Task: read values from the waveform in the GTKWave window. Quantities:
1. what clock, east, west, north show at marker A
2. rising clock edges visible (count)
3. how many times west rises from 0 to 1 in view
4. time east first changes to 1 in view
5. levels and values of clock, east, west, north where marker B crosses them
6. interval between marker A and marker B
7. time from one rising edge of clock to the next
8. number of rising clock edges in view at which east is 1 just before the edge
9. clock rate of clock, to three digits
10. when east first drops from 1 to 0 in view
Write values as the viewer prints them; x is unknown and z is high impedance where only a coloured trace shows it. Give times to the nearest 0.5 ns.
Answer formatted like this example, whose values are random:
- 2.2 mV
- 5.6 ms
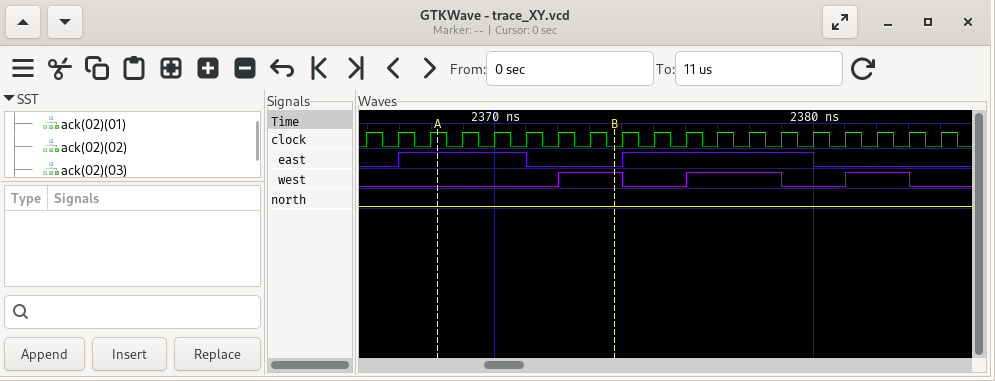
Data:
- clock=1, east=1, west=0, north=0
- 19
- 3
- 2367 ns
- clock=0, east=0, west=1, north=0
- 5.5 ns
- 1 ns
- 10
- 1.00 GHz
- 2371 ns
